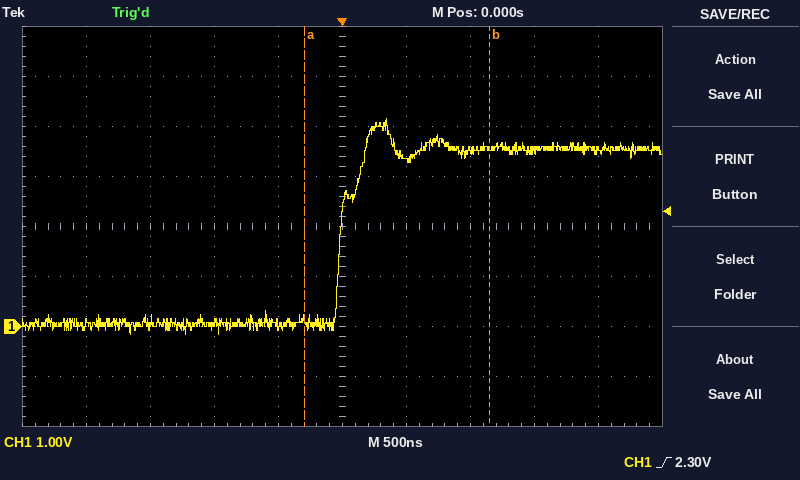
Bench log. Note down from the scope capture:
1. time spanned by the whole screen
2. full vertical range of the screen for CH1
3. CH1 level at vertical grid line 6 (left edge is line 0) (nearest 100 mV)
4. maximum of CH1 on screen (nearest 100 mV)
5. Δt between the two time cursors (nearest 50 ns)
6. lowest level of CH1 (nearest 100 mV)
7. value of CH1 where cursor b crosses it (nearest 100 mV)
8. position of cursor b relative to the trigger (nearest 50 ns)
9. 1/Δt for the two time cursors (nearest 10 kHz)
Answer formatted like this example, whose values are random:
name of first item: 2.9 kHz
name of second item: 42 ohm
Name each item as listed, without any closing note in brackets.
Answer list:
time spanned by the whole screen: 5 µs
full vertical range of the screen for CH1: 8 V
CH1 level at vertical grid line 6 (left edge is line 0): 3.3 V
maximum of CH1 on screen: 4.2 V
Δt between the two time cursors: 1.45 µs
lowest level of CH1: -200 mV
value of CH1 where cursor b crosses it: 3.6 V
position of cursor b relative to the trigger: +1.15 µs
1/Δt for the two time cursors: 690 kHz
